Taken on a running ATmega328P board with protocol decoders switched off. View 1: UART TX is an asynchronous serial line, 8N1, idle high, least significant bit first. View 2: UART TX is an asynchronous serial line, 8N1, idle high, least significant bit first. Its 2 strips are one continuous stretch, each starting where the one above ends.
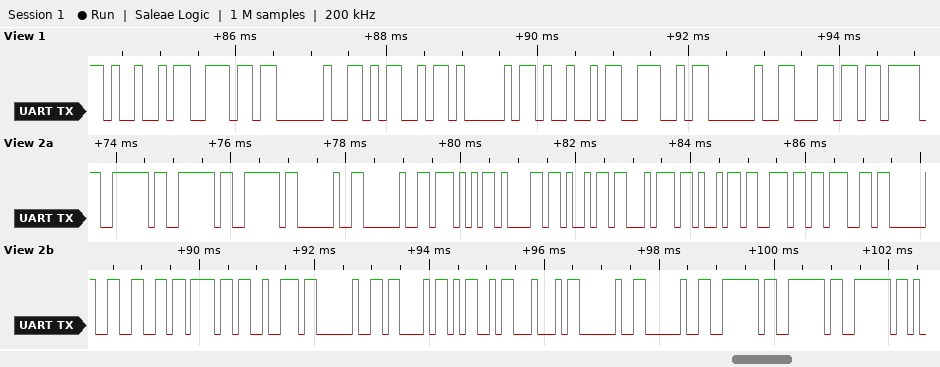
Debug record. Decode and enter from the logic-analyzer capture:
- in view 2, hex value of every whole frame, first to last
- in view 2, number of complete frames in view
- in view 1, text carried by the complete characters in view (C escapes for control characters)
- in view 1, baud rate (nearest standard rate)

0x7E 0x7E 0x7E 0x20 0x20 0x57 0x61 0x69 0x74 0x69 0x6E 0x67 0x20 0x66 0x6F 0x72 0x20 0x43 0x4D 0x44 0x20 0x20 0x7E 0x7E 0x7E
25
"In MAIN l"
9600 baud
